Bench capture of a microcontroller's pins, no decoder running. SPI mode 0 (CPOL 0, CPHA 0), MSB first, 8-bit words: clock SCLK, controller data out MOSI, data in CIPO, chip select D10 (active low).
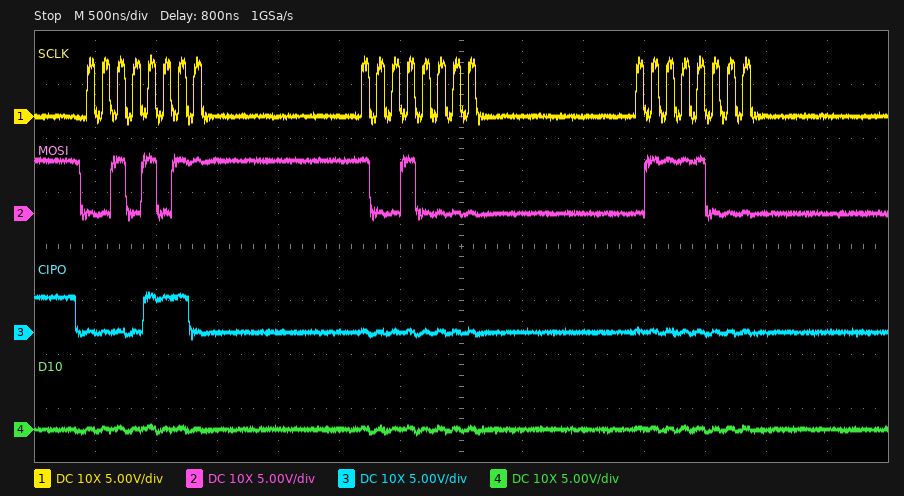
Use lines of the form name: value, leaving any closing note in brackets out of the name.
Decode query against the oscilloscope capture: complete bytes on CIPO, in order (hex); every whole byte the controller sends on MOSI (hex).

complete bytes on CIPO, in order: 0x0E 0x00 0x00
every whole byte the controller sends on MOSI: 0x2B 0x90 0x78
